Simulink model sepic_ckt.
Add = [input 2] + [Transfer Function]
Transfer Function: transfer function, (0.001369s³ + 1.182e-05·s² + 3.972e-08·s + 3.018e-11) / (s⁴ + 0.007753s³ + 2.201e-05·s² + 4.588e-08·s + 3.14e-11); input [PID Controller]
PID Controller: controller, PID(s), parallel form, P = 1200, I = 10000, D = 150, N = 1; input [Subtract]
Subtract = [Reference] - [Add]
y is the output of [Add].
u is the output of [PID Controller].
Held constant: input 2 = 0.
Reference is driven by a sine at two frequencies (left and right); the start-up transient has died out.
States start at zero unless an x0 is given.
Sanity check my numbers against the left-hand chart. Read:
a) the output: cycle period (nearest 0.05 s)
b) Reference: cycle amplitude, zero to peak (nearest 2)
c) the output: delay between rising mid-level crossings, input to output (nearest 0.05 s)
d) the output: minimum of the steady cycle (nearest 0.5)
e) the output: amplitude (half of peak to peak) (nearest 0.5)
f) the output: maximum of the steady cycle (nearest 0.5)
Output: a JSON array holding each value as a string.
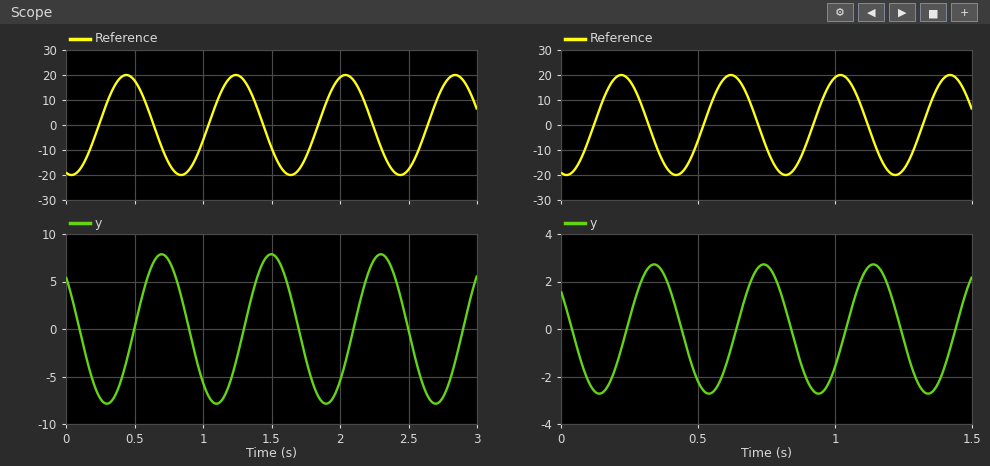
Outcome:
["0.80 s", "20", "0.25 s", "-8.0", "8.0", "8.0"]
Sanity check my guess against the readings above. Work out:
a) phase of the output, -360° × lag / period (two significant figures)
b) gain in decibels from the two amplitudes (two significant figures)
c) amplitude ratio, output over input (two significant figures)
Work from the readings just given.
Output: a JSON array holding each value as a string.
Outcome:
["-110°", "-8.0 dB", "0.40"]
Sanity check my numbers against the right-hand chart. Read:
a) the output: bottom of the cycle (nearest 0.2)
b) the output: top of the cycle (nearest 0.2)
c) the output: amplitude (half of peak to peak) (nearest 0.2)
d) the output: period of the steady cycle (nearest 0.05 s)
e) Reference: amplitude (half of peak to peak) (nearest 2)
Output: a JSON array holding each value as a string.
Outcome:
["-2.8", "2.8", "2.8", "0.40 s", "20"]
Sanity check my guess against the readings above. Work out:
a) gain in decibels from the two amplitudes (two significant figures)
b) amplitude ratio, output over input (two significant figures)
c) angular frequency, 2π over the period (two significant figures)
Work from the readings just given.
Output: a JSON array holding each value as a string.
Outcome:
["-17 dB", "0.14", "16 rad/s"]
